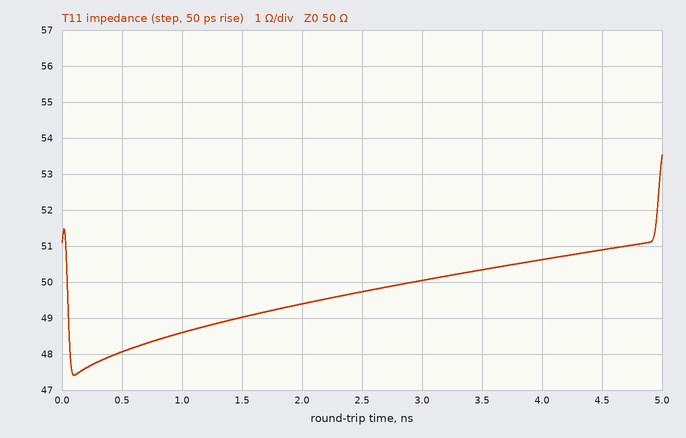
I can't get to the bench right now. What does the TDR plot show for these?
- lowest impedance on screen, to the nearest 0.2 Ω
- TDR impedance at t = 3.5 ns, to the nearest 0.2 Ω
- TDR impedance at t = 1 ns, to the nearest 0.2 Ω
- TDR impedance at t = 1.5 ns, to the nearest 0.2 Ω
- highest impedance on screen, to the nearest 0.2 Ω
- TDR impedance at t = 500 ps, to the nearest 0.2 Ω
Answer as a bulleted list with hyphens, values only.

- 47.4 Ω
- 50.4 Ω
- 48.6 Ω
- 49.0 Ω
- 53.6 Ω
- 48.0 Ω
